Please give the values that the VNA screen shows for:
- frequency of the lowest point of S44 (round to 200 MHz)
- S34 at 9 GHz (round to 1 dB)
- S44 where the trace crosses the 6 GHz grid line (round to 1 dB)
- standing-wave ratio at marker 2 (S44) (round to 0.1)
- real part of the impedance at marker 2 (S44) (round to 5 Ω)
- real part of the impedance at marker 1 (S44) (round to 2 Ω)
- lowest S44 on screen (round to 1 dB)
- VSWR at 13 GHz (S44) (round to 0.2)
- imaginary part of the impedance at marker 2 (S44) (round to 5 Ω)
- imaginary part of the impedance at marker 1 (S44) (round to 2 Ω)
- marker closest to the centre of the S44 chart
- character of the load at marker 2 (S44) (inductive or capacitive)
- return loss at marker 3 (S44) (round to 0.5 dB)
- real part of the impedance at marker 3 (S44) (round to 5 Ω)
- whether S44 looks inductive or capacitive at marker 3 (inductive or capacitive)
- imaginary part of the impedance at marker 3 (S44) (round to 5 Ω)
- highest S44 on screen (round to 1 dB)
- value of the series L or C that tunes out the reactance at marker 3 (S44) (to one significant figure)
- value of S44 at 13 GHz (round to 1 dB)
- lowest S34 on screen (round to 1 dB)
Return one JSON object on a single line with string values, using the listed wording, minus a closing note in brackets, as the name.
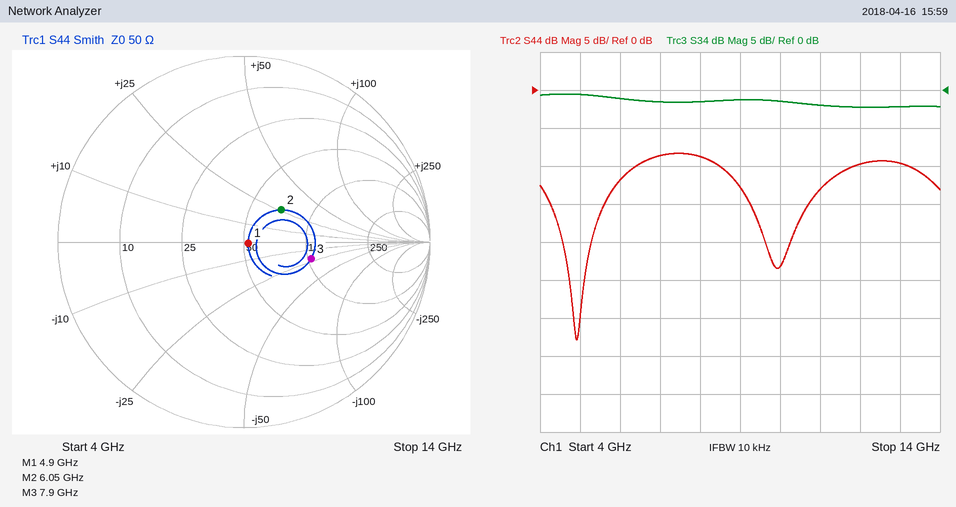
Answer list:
{"frequency of the lowest point of S44": "5.0 GHz", "S34 at 9 GHz": "-1 dB", "S44 where the trace crosses the 6 GHz grid line": "-12 dB", "standing-wave ratio at marker 2 (S44)": "1.7", "real part of the impedance at marker 2 (S44)": "70 Ω", "real part of the impedance at marker 1 (S44)": "52 Ω", "lowest S44 on screen": "-33 dB", "VSWR at 13 GHz (S44)": "2.0", "imaginary part of the impedance at marker 2 (S44)": "+25 Ω", "imaginary part of the impedance at marker 1 (S44)": "0 Ω", "marker closest to the centre of the S44 chart": "marker 1", "character of the load at marker 2 (S44)": "inductive", "return loss at marker 3 (S44)": "8.5 dB", "real part of the impedance at marker 3 (S44)": "105 Ω", "whether S44 looks inductive or capacitive at marker 3": "capacitive", "imaginary part of the impedance at marker 3 (S44)": "-20 Ω", "highest S44 on screen": "-8 dB", "value of the series L or C that tunes out the reactance at marker 3 (S44)": "400 pH", "value of S44 at 13 GHz": "-10 dB", "lowest S34 on screen": "-2 dB"}
